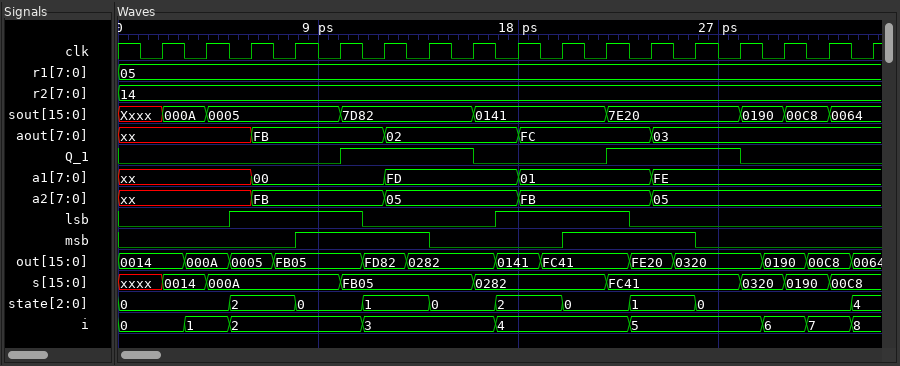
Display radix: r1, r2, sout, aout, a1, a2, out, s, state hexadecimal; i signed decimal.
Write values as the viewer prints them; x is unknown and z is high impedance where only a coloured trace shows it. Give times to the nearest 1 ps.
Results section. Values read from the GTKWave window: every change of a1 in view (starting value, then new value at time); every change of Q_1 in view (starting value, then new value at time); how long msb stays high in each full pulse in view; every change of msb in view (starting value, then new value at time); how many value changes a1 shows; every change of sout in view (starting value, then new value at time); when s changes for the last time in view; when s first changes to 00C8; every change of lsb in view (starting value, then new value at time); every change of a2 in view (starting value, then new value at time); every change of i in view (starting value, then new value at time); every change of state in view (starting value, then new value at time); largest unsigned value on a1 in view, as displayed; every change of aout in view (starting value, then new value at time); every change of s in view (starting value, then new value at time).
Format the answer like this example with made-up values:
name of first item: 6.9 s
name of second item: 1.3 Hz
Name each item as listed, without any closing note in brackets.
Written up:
every change of a1 in view: xx, 00 at 6 ps, FD at 12 ps, 01 at 18 ps, FE at 24 ps
every change of Q_1 in view: 0, 1 at 10 ps, 0 at 16 ps, 1 at 22 ps, 0 at 28 ps
how long msb stays high in each full pulse in view: 6 ps, 6 ps
every change of msb in view: 0, 1 at 8 ps, 0 at 14 ps, 1 at 20 ps, 0 at 26 ps
how many value changes a1 shows: 4
every change of sout in view: Xxxx, 000A at 2 ps, 0005 at 4 ps, 7D82 at 10 ps, 0141 at 16 ps, 7E20 at 22 ps, 0190 at 28 ps, 00C8 at 30 ps, 0064 at 32 ps
when s changes for the last time in view: 32 ps
when s first changes to 00C8: 32 ps
every change of lsb in view: 0, 1 at 5 ps, 0 at 11 ps, 1 at 17 ps, 0 at 23 ps
every change of a2 in view: xx, FB at 6 ps, 05 at 12 ps, FB at 18 ps, 05 at 24 ps
every change of i in view: 0, 1 at 3 ps, 2 at 5 ps, 3 at 11 ps, 4 at 17 ps, 5 at 23 ps, 6 at 29 ps, 7 at 31 ps, 8 at 33 ps
every change of state in view: 0, 2 at 5 ps, 0 at 8 ps, 1 at 11 ps, 0 at 14 ps, 2 at 17 ps, 0 at 20 ps, 1 at 23 ps, 0 at 26 ps, 4 at 33 ps
largest unsigned value on a1 in view, as displayed: FE
every change of aout in view: xx, FB at 6 ps, 02 at 12 ps, FC at 18 ps, 03 at 24 ps
every change of s in view: xxxx, 0014 at 2 ps, 000A at 4 ps, FB05 at 10 ps, 0282 at 16 ps, FC41 at 22 ps, 0320 at 28 ps, 0190 at 30 ps, 00C8 at 32 ps
